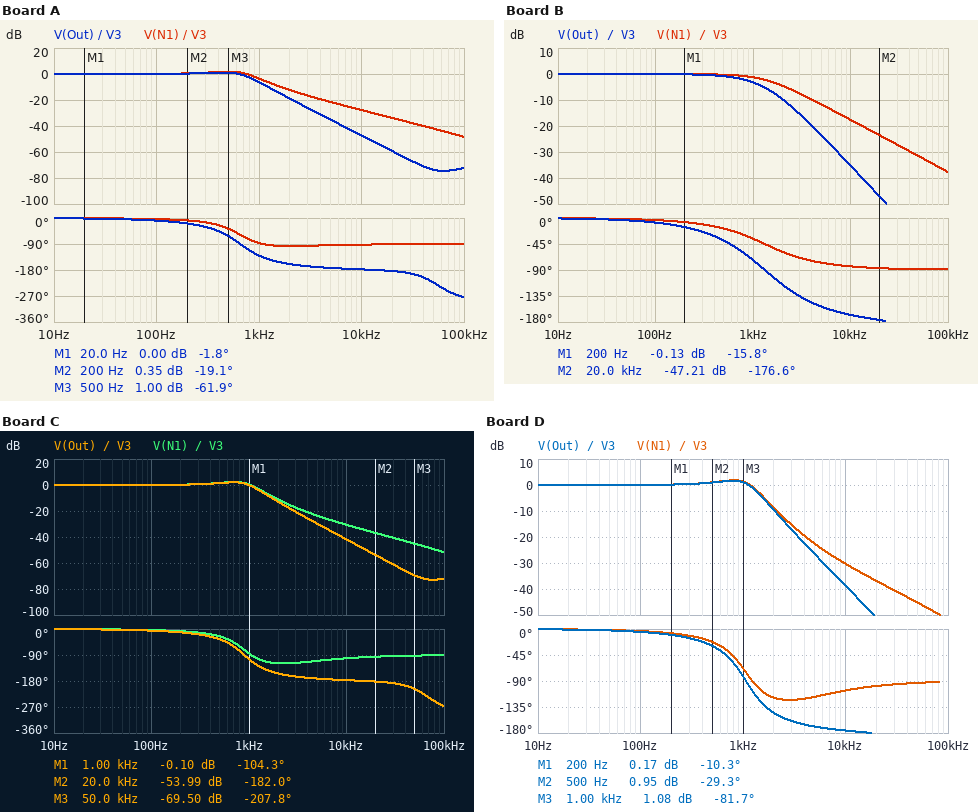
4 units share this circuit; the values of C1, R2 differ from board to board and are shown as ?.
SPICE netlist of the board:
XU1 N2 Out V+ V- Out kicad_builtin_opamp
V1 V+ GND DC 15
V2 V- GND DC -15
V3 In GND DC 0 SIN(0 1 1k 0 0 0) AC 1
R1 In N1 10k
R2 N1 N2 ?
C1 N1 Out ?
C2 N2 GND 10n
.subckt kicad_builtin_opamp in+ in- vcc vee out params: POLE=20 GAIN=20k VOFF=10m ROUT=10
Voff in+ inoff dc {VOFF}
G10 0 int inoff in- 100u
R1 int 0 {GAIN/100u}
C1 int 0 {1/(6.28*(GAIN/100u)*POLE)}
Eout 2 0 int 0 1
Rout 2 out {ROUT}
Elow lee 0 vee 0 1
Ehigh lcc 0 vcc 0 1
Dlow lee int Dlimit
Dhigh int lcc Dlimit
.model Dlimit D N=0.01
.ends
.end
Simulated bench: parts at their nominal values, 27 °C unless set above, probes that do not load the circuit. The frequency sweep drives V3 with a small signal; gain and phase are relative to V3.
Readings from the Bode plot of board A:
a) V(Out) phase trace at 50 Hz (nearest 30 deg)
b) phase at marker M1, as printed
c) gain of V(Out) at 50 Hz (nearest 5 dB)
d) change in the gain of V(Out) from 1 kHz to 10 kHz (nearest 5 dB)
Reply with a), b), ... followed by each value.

a) 0 deg
b) -1.8 deg
c) 0 dB
d) -40 dB
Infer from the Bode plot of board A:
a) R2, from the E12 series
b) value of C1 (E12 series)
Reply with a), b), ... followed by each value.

a) 15 kΩ
b) 39 nF
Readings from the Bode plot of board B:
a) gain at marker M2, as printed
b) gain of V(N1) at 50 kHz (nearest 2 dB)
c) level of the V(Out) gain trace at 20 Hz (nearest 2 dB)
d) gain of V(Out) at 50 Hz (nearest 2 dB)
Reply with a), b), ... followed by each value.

a) -47.21 dB
b) -32 dB
c) 0 dB
d) 0 dB
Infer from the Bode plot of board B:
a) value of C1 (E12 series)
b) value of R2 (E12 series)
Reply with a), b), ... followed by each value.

a) 12 nF
b) 12 kΩ
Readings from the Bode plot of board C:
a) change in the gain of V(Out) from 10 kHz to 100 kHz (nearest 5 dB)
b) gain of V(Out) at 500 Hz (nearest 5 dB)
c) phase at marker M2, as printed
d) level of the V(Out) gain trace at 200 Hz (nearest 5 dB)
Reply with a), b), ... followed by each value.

a) -30 dB
b) 0 dB
c) -182.0 deg
d) 0 dB
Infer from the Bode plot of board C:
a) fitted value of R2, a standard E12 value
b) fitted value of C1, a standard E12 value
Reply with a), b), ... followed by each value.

a) 5.6 kΩ
b) 56 nF
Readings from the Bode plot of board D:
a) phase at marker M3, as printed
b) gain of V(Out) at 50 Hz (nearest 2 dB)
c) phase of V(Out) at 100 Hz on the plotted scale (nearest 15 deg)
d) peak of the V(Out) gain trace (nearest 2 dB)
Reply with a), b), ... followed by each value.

a) -81.7 deg
b) 0 dB
c) 0 deg
d) 2 dB
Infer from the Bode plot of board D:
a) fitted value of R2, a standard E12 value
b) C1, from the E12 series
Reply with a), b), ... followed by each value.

a) 3.9 kΩ
b) 56 nF
